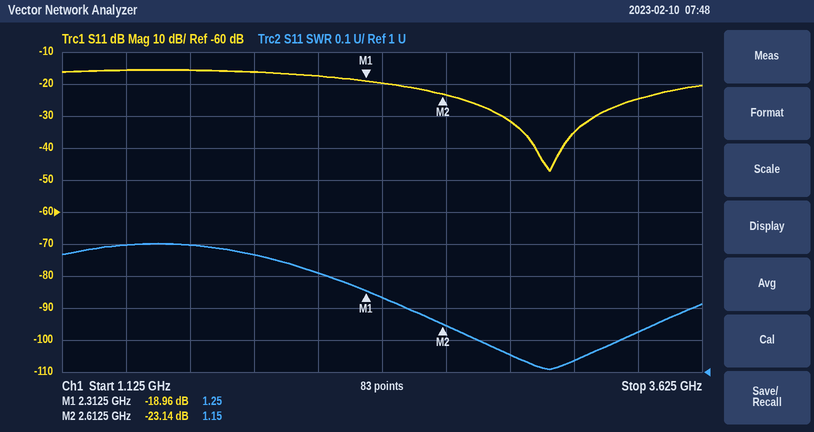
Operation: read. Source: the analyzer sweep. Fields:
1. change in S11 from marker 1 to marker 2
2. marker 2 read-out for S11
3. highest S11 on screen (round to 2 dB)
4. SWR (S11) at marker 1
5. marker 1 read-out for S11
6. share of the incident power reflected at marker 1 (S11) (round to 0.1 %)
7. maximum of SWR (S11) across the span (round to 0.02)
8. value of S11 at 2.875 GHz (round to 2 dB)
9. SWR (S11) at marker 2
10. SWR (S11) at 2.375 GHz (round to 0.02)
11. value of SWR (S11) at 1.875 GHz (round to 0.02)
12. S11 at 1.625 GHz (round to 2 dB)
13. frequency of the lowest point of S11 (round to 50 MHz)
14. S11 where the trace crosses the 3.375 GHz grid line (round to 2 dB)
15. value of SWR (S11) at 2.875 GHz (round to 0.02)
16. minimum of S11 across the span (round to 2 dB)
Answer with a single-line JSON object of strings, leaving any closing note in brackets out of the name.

{"change in S11 from marker 1 to marker 2": "-4.18 dB", "marker 2 read-out for S11": "-23.14 dB", "highest S11 on screen": "-16 dB", "SWR (S11) at marker 1": "1.25", "marker 1 read-out for S11": "-18.96 dB", "share of the incident power reflected at marker 1 (S11)": "1.3 %", "maximum of SWR (S11) across the span": "1.40", "value of S11 at 2.875 GHz": "-32 dB", "SWR (S11) at marker 2": "1.15", "SWR (S11) at 2.375 GHz": "1.24", "value of SWR (S11) at 1.875 GHz": "1.36", "S11 at 1.625 GHz": "-16 dB", "frequency of the lowest point of S11": "3.05 GHz", "S11 where the trace crosses the 3.375 GHz grid line": "-24 dB", "value of SWR (S11) at 2.875 GHz": "1.06", "minimum of S11 across the span": "-48 dB"}
